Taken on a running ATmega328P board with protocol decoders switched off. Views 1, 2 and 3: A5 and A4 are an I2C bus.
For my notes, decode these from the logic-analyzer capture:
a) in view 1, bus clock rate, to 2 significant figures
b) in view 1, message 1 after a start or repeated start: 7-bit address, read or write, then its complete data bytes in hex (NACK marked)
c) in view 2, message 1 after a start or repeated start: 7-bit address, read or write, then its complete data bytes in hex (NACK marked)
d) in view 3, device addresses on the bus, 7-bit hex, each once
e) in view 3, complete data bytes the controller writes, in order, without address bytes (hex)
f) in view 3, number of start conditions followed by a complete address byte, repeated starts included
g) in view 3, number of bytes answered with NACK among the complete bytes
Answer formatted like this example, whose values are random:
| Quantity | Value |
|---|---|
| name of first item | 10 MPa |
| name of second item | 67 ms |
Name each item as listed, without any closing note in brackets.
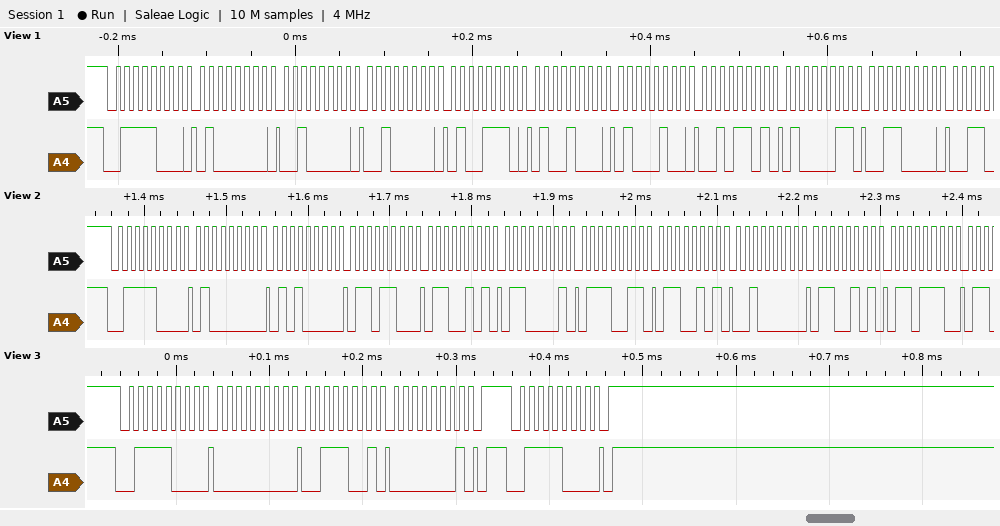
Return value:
| Quantity | Value |
|---|---|
| in view 1, bus clock rate, to 2 significant figures | 100 kHz |
| in view 1, message 1 after a start or repeated start: 7-bit address, read or write, then its complete data bytes in hex | 0x3C write: 40 20 20 4E 48 44 2D 43 30 |
| in view 2, message 1 after a start or repeated start: 7-bit address, read or write, then its complete data bytes in hex | 0x3C write: 40 50 6C 65 61 73 65 20 65 6E |
| in view 3, device addresses on the bus, 7-bit hex, each once | 0x3C |
| in view 3, complete data bytes the controller writes, in order, without address bytes | 00 39 01 |
| in view 3, number of start conditions followed by a complete address byte, repeated starts included | 2 |
| in view 3, number of bytes answered with NACK among the complete bytes | 0 |
